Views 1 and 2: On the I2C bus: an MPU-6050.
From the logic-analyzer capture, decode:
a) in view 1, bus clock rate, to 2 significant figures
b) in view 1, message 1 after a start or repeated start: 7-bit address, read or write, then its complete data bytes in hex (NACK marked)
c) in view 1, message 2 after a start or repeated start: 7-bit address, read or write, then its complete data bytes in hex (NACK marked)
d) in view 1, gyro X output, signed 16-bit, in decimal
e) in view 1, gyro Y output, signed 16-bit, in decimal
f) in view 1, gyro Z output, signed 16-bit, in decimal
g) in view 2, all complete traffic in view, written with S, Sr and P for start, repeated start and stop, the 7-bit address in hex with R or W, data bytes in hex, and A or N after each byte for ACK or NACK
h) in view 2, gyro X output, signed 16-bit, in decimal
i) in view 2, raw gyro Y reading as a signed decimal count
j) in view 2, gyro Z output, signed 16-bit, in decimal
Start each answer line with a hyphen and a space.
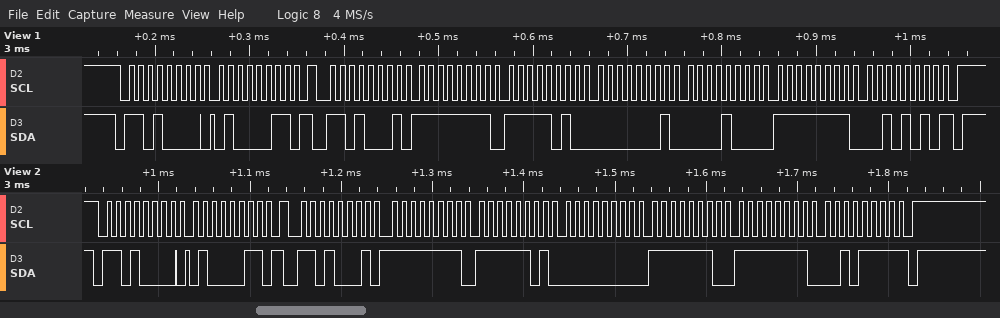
- 100 kHz
- 0x68 write: 43
- 0x68 read: FF FA 01 08 FF 2A NACK
- -6
- 264
- -214
- S 68W A 43 A Sr 68R A FF A FD A 00 A FE A FF A 2F N P
- -3
- 254
- -209
